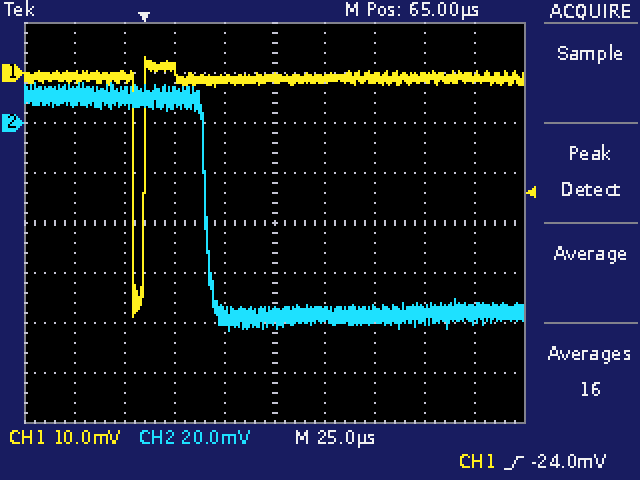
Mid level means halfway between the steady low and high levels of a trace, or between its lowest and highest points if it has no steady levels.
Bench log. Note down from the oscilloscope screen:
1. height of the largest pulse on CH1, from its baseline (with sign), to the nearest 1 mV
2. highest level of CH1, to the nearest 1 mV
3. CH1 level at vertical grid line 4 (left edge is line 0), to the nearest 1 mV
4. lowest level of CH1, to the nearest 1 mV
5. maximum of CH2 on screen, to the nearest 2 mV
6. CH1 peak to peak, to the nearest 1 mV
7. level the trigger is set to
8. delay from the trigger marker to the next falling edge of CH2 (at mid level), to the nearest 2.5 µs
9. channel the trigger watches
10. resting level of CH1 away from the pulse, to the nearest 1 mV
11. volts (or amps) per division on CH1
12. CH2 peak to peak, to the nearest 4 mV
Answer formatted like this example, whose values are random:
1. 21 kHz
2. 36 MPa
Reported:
1. -48 mV
2. 3 mV
3. -1 mV
4. -49 mV
5. 16 mV
6. 52 mV
7. -24.0 mV
8. 30.0 µs
9. CH1
10. -1 mV
11. 10 mV
12. 100 mV
